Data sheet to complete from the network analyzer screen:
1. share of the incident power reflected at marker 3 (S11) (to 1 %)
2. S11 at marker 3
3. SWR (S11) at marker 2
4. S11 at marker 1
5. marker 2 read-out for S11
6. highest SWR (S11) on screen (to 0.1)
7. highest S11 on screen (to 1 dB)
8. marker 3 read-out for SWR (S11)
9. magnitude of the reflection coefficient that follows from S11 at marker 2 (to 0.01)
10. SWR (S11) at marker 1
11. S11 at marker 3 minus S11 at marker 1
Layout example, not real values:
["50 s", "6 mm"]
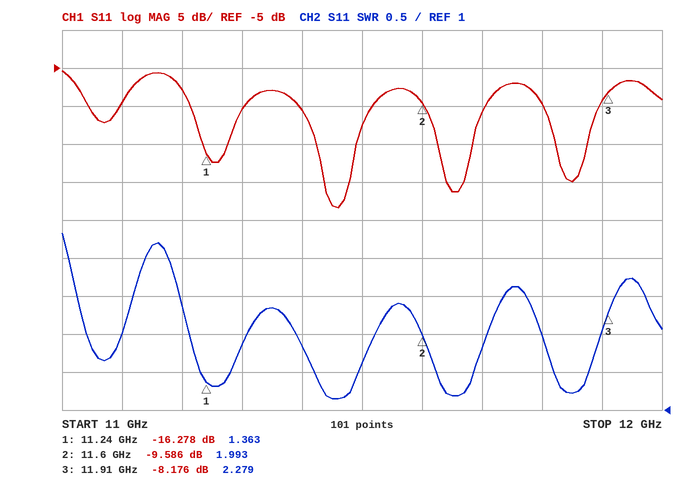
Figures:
["15 %", "-8.176 dB", "1.993", "-16.278 dB", "-9.586 dB", "3.3", "-5 dB", "2.279", "0.33", "1.363", "8.102 dB"]
